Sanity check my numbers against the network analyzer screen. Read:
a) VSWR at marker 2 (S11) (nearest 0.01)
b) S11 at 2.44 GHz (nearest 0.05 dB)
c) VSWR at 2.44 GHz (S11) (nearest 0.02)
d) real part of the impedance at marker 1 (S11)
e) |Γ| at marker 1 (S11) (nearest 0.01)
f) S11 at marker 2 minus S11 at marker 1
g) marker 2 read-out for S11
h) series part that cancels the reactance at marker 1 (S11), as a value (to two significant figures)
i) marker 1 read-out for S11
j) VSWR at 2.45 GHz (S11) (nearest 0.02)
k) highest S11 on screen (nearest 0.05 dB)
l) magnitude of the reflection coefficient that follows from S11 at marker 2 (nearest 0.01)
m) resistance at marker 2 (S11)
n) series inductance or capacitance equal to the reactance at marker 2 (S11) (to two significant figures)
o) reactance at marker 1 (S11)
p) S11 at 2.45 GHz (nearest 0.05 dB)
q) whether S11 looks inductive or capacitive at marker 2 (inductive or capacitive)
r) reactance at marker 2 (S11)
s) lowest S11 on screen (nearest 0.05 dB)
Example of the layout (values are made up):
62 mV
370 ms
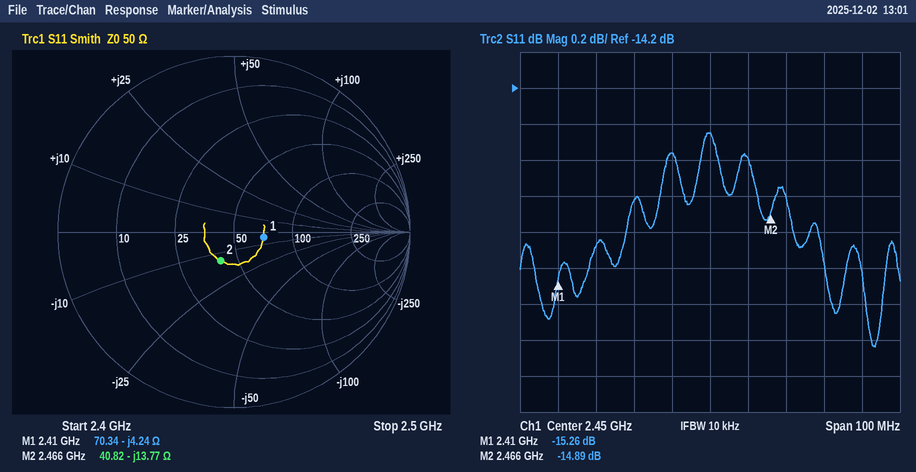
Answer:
1.44
-14.55 dB
1.46
70.34 Ω
0.17
0.37 dB
-14.89 dB
280 pH
-15.26 dB
1.46
-14.45 dB
0.18
40.82 Ω
4.7 pF
-4.24 Ω
-14.45 dB
capacitive
-13.77 Ω
-15.65 dB
